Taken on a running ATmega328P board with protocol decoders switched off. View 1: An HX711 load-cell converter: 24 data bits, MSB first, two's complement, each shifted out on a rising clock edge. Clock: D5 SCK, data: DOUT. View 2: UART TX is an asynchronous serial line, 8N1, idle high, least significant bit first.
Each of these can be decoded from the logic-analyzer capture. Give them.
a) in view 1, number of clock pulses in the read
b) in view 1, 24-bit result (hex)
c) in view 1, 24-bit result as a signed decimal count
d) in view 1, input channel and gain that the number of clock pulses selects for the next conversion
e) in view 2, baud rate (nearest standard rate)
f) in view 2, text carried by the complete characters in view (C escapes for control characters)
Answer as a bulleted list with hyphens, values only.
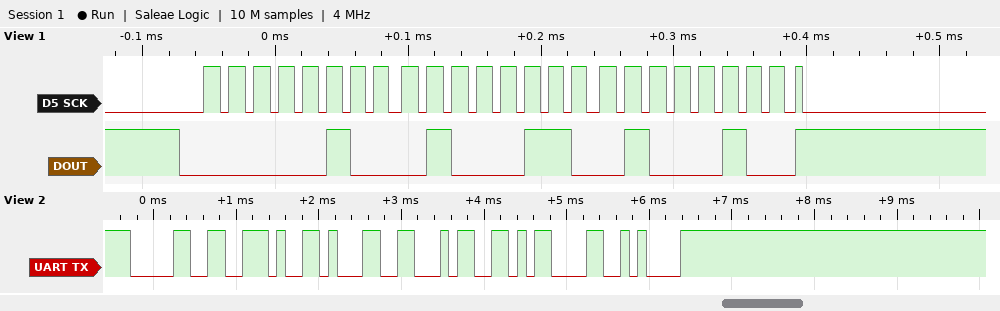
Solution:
- 25
- 0x044644
- 280132
- channel A, gain 128
- 9600 baud
- "0.14\r\n"
